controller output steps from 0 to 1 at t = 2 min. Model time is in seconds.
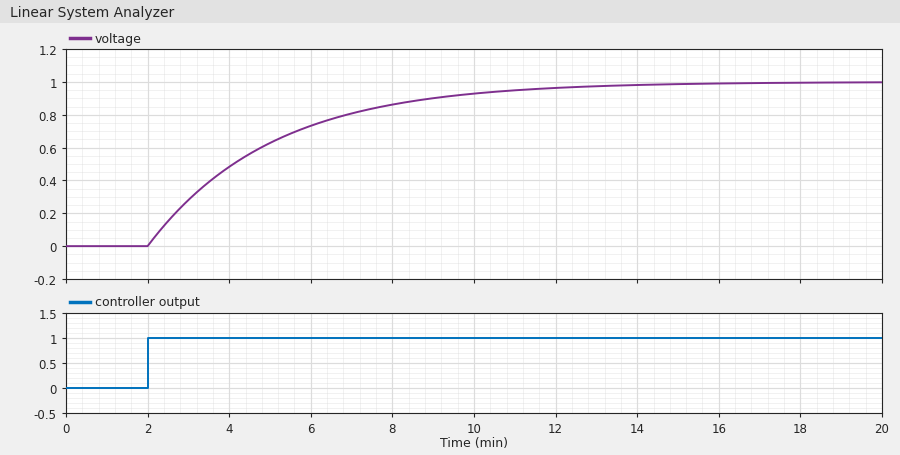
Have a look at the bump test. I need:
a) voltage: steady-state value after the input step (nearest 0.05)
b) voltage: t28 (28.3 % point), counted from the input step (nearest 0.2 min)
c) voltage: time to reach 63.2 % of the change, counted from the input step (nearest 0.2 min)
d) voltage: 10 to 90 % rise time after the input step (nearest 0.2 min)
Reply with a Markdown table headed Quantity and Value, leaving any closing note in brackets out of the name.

| Quantity | Value |
|---|---|
| voltage: steady-state value after the input step | 1.00 |
| voltage: t28 (28.3 % point), counted from the input step | 1.0 min |
| voltage: time to reach 63.2 % of the change, counted from the input step | 3.0 min |
| voltage: 10 to 90 % rise time after the input step | 6.6 min |
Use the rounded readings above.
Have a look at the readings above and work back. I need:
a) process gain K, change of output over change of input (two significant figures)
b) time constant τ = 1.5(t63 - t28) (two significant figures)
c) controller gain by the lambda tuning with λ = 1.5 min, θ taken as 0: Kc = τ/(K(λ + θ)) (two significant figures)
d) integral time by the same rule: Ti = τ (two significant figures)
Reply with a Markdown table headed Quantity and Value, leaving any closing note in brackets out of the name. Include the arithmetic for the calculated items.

| Quantity | Value |
|---|---|
| process gain K, change of output over change of input | (1 - 0) / 1 = 1.0 |
| time constant τ = 1.5(t63 - t28) | 1.5 × (3 - 1) = 3.0 min |
| controller gain by the lambda tuning with λ = 1.5 min, θ taken as 0: Kc = τ/(K(λ + θ)) | 3 / (1 × (1.5 + 0)) = 2.0 |
| integral time by the same rule: Ti = τ | 3.0 min |
